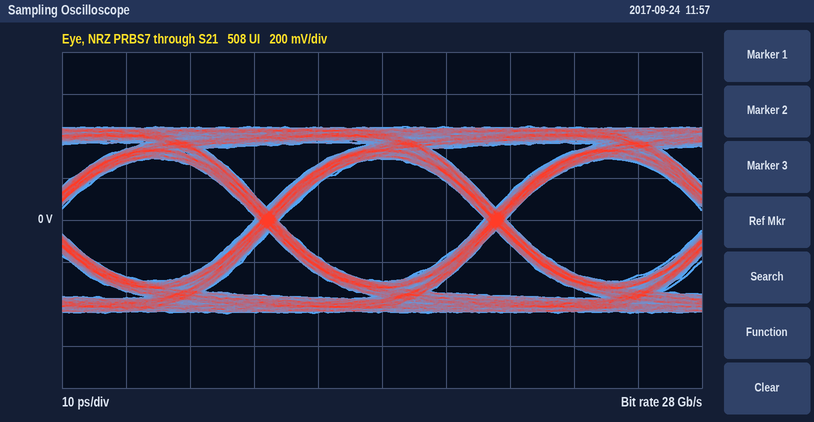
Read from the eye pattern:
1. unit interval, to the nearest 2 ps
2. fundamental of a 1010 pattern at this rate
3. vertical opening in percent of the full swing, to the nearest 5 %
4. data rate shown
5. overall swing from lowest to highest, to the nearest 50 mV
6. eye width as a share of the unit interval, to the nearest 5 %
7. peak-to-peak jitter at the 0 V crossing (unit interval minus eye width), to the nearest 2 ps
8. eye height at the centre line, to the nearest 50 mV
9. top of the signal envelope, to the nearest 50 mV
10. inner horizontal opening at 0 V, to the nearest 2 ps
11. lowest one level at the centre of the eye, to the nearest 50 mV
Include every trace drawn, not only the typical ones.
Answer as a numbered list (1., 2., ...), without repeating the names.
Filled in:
1. 36 ps
2. 14 GHz
3. 65 %
4. 28 Gb/s
5. 900 mV
6. 90 %
7. 4 ps
8. 600 mV
9. 450 mV
10. 32 ps
11. 300 mV
